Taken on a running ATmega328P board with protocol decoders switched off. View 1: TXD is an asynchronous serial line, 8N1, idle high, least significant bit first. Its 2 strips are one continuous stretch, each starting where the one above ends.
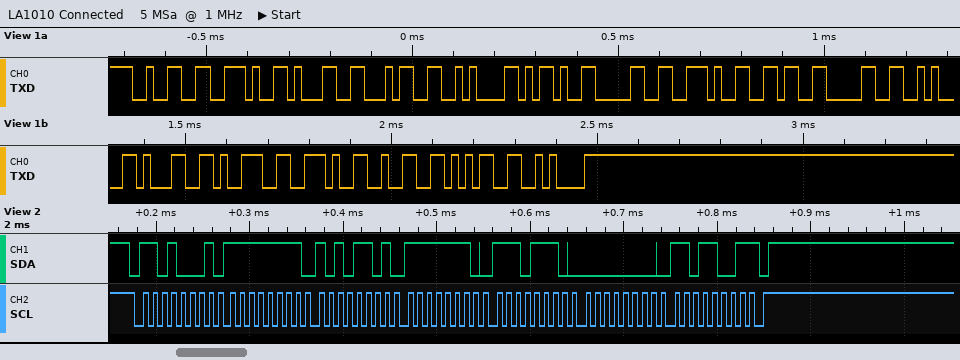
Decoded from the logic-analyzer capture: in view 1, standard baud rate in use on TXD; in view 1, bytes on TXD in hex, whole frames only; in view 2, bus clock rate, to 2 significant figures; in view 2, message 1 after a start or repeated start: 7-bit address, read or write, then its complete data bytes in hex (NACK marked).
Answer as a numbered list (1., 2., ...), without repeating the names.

1. 57600 baud
2. 32 2E 31 34 0A 2D 30 2E 36 30 0A 31 39 2E 32 35 0A
3. 100 kHz
4. 0x68 read: FF AD FE EE 00 D9 NACK
